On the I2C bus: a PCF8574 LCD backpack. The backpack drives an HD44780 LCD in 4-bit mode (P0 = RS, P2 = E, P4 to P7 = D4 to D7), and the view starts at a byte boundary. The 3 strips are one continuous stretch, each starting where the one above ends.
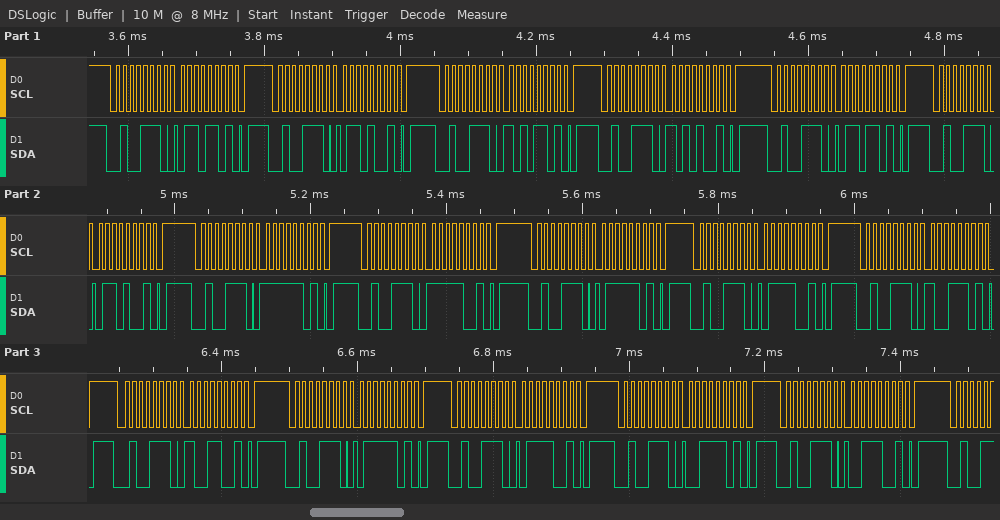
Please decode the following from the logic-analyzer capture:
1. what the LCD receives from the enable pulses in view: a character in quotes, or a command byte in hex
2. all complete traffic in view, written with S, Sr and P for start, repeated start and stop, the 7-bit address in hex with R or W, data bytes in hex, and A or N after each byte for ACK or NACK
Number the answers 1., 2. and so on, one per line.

1. 'j' 'o' 'y' 's'
2. S 27W A 6D A P S 27W A 69 A P S 27W A AD A P S 27W A A9 A P S 27W A 6D A P S 27W A 69 A P S 27W A FD A P S 27W A F9 A P S 27W A 7D A P S 27W A 79 A P S 27W A 9D A P S 27W A 99 A P S 27W A 7D A P S 27W A 79 A P S 27W A 3D A P S 27W A 39 A P
